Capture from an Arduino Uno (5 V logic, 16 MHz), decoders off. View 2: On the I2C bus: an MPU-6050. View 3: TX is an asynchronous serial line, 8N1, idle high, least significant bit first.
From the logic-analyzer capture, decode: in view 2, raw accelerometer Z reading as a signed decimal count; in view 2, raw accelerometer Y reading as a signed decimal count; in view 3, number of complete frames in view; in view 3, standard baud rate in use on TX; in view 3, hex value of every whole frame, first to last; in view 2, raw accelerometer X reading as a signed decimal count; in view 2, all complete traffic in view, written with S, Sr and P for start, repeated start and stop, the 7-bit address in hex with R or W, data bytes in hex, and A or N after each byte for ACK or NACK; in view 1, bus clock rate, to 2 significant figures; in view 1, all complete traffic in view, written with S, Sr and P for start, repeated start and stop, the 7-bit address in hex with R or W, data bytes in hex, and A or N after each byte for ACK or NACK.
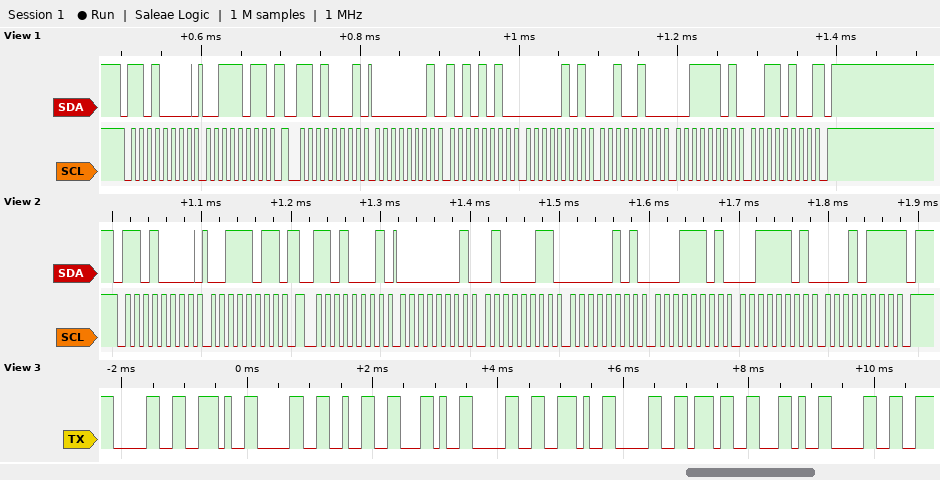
15639
1309
11
9600 baud
30 2E 30 32 2C 30 2E 30 37 2C 30
323
S 68W A 3B A Sr 68R A 01 A 43 A 05 A 1D A 3D A 17 N P
100 kHz
S 68W A 3B A Sr 68R A 01 A AA A 05 A 24 A 3D A 34 N P
